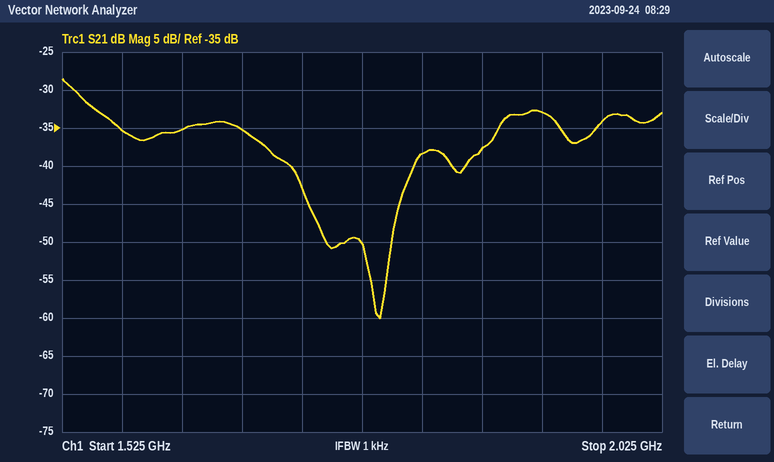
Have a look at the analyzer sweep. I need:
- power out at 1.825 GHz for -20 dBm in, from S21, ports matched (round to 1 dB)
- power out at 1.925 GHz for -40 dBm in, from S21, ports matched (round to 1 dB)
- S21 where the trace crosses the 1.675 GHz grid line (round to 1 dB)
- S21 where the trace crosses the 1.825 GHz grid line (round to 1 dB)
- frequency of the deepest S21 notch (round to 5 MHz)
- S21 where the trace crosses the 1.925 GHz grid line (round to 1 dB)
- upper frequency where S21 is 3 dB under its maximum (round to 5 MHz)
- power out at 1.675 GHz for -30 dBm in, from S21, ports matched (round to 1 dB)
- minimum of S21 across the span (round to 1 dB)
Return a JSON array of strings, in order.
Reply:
["-58 dBm", "-73 dBm", "-35 dB", "-38 dB", "1.790 GHz", "-33 dB", "1.545 GHz", "-65 dBm", "-60 dB"]
